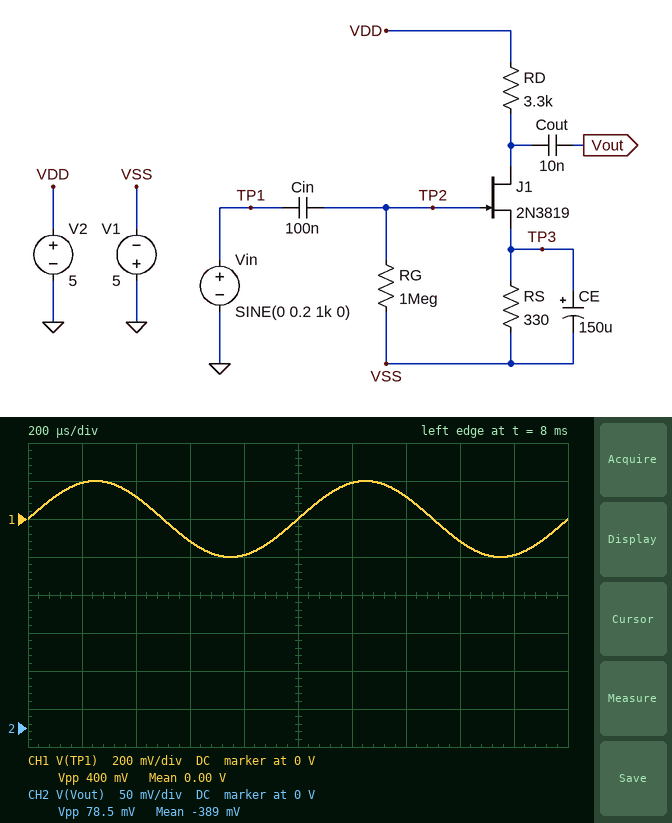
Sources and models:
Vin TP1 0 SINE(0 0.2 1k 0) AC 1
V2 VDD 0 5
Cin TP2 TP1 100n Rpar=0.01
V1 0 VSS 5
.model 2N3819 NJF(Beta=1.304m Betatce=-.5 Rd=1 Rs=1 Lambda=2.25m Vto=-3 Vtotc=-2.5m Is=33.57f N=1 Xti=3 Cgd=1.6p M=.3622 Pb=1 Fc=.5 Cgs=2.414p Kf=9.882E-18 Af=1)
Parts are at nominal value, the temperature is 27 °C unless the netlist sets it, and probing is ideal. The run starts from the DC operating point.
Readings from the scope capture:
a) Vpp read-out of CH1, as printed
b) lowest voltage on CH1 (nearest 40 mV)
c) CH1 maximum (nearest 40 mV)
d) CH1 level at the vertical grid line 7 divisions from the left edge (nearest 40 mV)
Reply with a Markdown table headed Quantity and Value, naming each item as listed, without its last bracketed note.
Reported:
| Quantity | Value |
|---|---|
| Vpp read-out of CH1, as printed | 400 mV |
| lowest voltage on CH1 | -200 mV |
| CH1 maximum | 200 mV |
| CH1 level at the vertical grid line 7 divisions from the left edge | 120 mV |
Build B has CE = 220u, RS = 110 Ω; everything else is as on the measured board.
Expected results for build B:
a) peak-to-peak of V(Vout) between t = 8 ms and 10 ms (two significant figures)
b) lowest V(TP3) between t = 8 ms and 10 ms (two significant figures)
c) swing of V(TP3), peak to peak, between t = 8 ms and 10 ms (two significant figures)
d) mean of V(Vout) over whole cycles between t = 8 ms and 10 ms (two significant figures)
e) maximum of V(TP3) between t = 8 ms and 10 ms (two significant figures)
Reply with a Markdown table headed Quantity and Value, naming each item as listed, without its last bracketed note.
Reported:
| Quantity | Value |
|---|---|
| peak-to-peak of V(Vout) between t = 8 ms and 10 ms | 170 mV |
| lowest V(TP3) between t = 8 ms and 10 ms | -730 mV |
| swing of V(TP3), peak to peak, between t = 8 ms and 10 ms | 93 mV |
| mean of V(Vout) over whole cycles between t = 8 ms and 10 ms | -460 mV |
| maximum of V(TP3) between t = 8 ms and 10 ms | -640 mV |
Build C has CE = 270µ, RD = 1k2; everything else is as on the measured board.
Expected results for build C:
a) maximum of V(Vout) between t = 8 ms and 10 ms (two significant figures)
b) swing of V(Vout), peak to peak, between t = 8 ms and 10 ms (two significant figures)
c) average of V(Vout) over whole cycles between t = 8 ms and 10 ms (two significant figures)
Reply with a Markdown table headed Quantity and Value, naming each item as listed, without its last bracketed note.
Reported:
| Quantity | Value |
|---|---|
| maximum of V(Vout) between t = 8 ms and 10 ms | -45 mV |
| swing of V(Vout), peak to peak, between t = 8 ms and 10 ms | 51 mV |
| average of V(Vout) over whole cycles between t = 8 ms and 10 ms | -65 mV |
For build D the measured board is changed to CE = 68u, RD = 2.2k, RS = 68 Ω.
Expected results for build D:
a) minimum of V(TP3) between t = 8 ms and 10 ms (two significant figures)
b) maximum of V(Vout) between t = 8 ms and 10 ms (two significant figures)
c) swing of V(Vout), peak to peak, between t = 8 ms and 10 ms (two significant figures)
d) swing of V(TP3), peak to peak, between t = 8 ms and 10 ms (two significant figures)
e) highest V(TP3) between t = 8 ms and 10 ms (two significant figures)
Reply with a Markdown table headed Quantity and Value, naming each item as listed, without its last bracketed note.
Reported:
| Quantity | Value |
|---|---|
| minimum of V(TP3) between t = 8 ms and 10 ms | -940 mV |
| maximum of V(Vout) between t = 8 ms and 10 ms | -280 mV |
| swing of V(Vout), peak to peak, between t = 8 ms and 10 ms | 340 mV |
| swing of V(TP3), peak to peak, between t = 8 ms and 10 ms | 320 mV |
| highest V(TP3) between t = 8 ms and 10 ms | -620 mV |
